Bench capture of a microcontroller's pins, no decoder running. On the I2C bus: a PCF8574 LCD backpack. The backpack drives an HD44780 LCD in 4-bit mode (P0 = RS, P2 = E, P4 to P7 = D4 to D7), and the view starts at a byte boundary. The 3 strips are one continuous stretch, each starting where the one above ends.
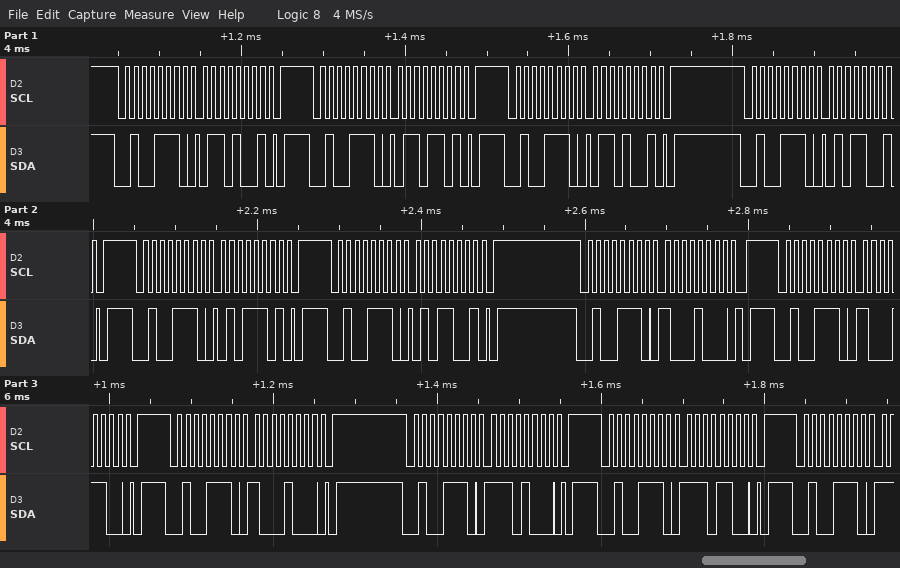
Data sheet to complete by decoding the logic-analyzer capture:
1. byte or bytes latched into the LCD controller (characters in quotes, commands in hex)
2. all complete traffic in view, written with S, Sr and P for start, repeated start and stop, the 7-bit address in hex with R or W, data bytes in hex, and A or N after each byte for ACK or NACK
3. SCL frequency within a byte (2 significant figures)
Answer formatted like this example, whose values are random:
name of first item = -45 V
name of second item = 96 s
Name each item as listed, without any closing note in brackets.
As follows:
byte or bytes latched into the LCD controller = 'e'
all complete traffic in view, written with S, Sr and P for start, repeated start and stop, the 7-bit address in hex with R or W, data bytes in hex, and A or N after each byte for ACK or NACK = S 27W A 69 A P S 27W A 6D A P S 27W A 69 A P S 27W A 59 A P S 27W A 5D A P S 27W A 59 A P S 27W A 88 A P S 27W A 8C A P S 27W A 88 A P S 27W A E8 A P S 27W A EC A P S 27W A
SCL frequency within a byte = 100 kHz
